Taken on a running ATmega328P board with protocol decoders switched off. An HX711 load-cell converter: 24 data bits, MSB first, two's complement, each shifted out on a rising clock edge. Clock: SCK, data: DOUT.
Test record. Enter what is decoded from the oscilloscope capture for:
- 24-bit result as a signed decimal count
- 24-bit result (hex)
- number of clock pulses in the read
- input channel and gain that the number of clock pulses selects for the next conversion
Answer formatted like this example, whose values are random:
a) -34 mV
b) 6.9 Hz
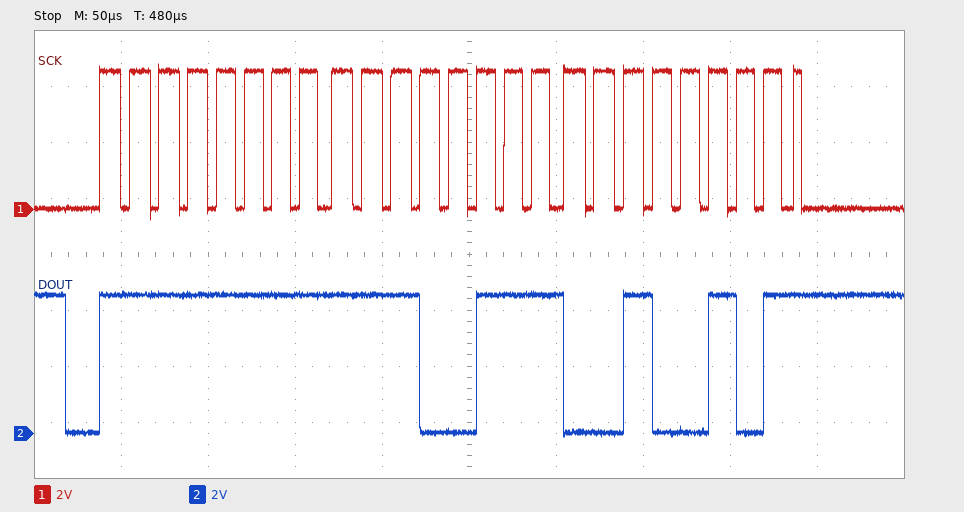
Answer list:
a) -6363
b) 0xFFE725
c) 25
d) channel A, gain 128
